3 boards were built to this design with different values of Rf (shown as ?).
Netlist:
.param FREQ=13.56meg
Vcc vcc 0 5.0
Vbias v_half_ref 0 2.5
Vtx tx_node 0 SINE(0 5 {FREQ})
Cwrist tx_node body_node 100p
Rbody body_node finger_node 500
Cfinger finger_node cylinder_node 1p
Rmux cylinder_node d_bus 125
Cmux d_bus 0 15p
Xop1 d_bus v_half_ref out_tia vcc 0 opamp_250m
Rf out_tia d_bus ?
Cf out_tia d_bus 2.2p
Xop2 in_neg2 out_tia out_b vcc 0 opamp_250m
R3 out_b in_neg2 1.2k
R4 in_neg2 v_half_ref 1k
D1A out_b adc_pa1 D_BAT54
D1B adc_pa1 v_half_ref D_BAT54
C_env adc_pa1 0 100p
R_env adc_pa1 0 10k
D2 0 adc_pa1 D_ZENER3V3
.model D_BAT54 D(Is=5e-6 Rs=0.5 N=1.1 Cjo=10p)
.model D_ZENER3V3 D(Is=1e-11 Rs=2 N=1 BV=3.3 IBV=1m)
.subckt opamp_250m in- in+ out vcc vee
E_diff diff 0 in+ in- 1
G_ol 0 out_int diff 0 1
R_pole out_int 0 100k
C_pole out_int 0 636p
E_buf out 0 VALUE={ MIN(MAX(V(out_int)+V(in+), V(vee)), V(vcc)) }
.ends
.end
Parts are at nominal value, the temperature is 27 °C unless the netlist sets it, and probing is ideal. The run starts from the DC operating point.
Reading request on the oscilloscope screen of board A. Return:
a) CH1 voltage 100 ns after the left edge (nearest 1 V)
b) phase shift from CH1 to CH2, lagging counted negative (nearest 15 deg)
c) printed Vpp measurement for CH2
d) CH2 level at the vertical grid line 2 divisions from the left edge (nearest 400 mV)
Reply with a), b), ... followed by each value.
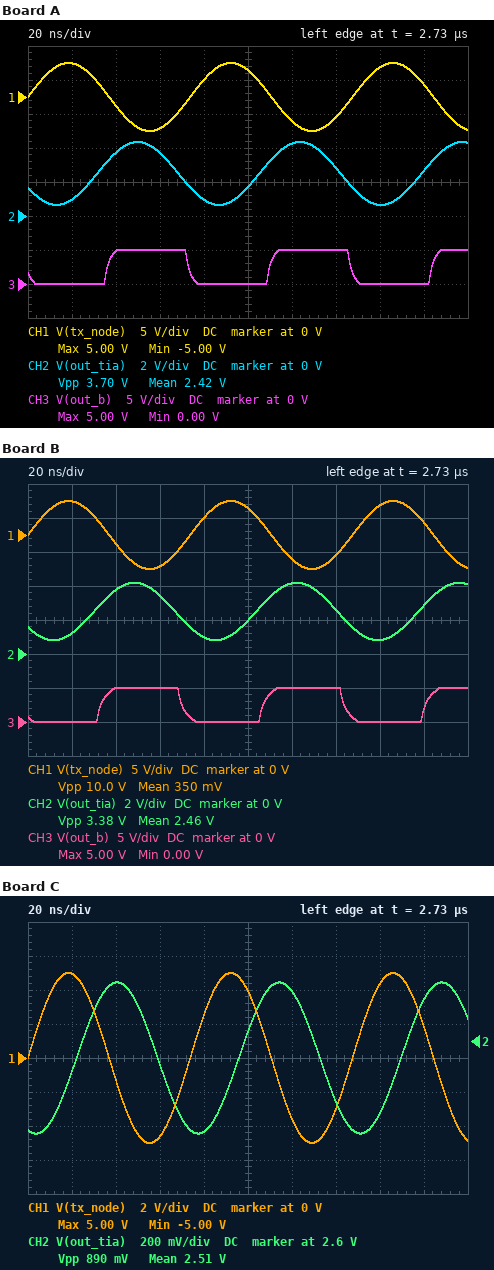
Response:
a) 4 V
b) -150 deg
c) 3.70 V
d) 3.6 V
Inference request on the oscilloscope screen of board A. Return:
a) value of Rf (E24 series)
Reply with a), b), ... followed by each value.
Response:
a) 5.1 kΩ
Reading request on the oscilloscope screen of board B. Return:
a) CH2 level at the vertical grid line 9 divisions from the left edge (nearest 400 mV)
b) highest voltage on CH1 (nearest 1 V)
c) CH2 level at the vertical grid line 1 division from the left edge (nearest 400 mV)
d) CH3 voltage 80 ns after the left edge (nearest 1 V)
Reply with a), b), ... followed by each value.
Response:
a) 2.8 V
b) 5 V
c) 1.2 V
d) 0 V
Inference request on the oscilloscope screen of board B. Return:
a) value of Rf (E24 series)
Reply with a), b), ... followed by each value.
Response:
a) 4.3 kΩ
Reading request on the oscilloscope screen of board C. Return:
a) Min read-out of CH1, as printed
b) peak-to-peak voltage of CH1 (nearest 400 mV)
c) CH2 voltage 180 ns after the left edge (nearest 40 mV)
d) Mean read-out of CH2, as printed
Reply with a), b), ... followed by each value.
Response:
a) -5.00 V
b) 10.0 V
c) 2.84 V
d) 2.51 V
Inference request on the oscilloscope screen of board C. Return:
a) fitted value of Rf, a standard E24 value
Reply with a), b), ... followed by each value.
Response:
a) 1 kΩ
